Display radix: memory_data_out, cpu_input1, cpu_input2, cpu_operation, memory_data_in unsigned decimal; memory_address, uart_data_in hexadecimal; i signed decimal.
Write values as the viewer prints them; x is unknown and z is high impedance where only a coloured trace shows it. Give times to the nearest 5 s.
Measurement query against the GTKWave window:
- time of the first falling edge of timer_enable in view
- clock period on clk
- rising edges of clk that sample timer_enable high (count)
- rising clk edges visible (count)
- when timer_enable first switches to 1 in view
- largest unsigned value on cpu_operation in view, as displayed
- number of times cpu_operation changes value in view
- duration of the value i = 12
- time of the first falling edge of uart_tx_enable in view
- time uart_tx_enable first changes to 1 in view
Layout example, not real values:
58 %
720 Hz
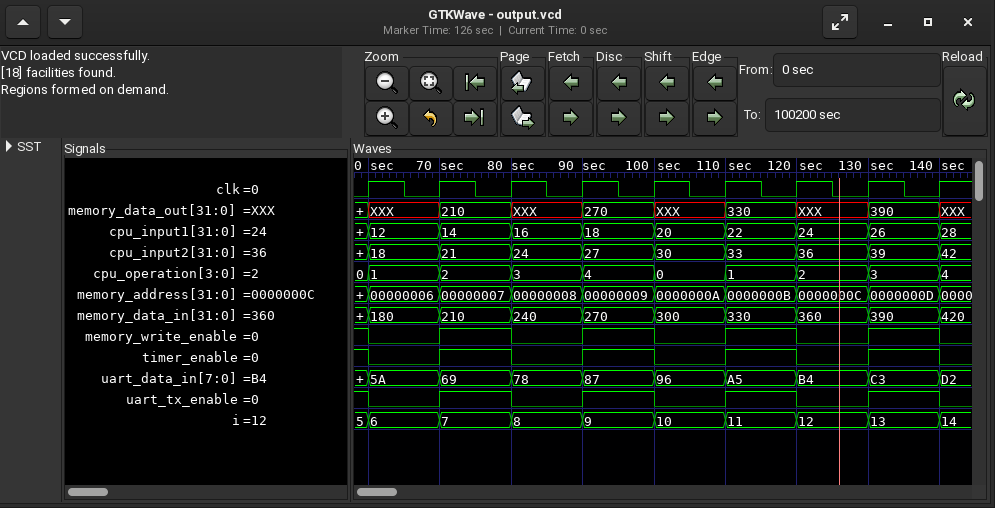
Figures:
60 s
10 s
5
9
70 s
4
9
10 s
60 s
70 s
